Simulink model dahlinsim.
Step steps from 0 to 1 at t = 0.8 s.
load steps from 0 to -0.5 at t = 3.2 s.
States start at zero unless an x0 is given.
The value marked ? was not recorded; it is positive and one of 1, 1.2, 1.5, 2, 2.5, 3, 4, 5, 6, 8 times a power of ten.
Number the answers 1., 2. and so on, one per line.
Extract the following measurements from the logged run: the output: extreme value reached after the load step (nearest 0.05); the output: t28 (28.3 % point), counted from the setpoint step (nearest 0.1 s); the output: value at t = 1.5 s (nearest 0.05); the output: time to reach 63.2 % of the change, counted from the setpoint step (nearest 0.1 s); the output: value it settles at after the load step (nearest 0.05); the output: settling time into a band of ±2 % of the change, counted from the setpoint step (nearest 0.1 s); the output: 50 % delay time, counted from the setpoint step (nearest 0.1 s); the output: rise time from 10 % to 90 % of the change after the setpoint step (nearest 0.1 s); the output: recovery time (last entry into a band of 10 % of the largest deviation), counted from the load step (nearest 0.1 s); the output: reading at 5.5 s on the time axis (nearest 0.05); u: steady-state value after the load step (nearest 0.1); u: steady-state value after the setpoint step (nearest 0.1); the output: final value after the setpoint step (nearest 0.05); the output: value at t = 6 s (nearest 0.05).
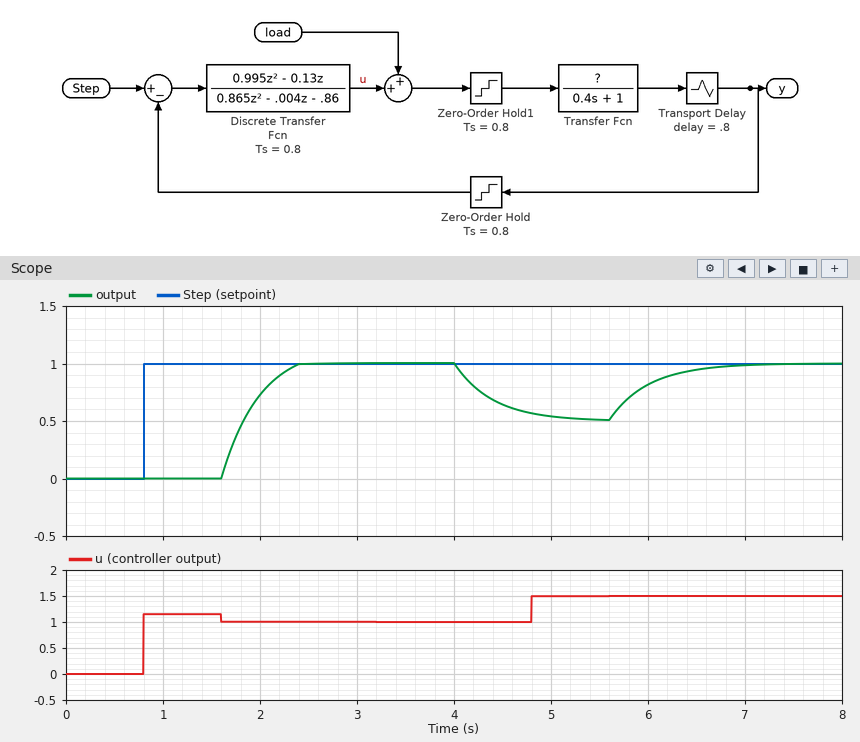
1. 0.50
2. 0.9 s
3. 0.00
4. 1.1 s
5. 1.00
6. 1.6 s
7. 1.0 s
8. 0.6 s
9. 3.3 s
10. 0.50
11. 1.5
12. 1.0
13. 1.00
14. 0.80
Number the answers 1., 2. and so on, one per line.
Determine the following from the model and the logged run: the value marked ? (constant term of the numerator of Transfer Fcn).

1. 1
